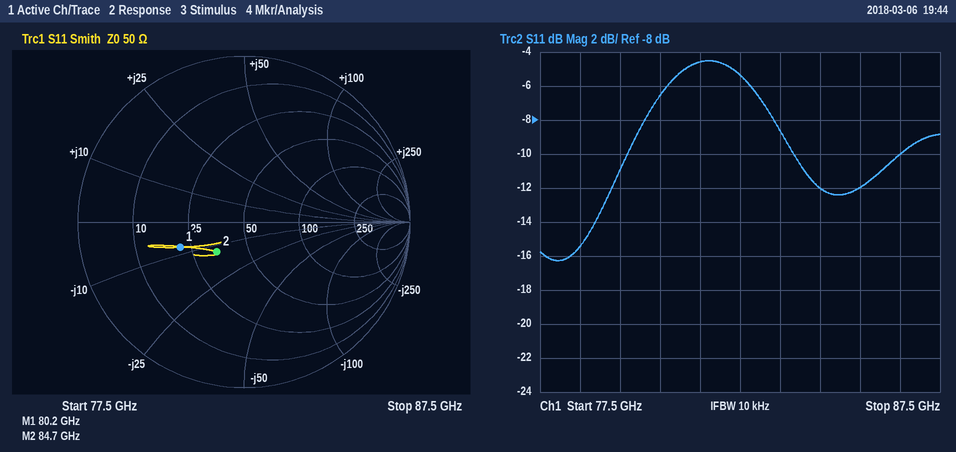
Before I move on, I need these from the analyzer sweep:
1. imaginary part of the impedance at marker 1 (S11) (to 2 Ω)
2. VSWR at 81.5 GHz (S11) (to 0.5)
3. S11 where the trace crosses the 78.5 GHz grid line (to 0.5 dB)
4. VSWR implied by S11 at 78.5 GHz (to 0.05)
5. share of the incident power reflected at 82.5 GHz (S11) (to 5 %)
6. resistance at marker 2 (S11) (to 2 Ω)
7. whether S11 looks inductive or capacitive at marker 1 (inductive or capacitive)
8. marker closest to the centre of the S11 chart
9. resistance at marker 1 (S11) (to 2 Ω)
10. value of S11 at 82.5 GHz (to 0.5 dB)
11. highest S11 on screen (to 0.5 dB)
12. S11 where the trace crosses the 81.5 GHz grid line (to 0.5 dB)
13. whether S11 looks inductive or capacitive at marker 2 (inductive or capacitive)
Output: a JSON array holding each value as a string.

["-8 Ω", "4.0", "-15.5 dB", "1.40", "30 %", "34 Ω", "capacitive", "marker 2", "22 Ω", "-5.5 dB", "-4.5 dB", "-4.5 dB", "capacitive"]
